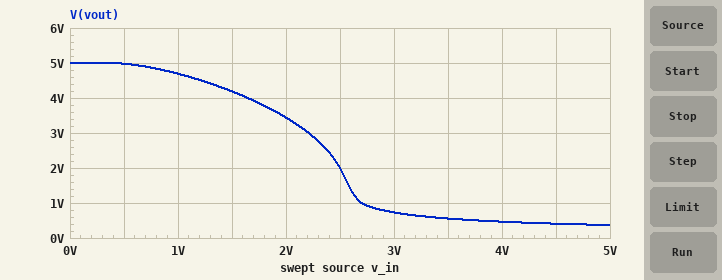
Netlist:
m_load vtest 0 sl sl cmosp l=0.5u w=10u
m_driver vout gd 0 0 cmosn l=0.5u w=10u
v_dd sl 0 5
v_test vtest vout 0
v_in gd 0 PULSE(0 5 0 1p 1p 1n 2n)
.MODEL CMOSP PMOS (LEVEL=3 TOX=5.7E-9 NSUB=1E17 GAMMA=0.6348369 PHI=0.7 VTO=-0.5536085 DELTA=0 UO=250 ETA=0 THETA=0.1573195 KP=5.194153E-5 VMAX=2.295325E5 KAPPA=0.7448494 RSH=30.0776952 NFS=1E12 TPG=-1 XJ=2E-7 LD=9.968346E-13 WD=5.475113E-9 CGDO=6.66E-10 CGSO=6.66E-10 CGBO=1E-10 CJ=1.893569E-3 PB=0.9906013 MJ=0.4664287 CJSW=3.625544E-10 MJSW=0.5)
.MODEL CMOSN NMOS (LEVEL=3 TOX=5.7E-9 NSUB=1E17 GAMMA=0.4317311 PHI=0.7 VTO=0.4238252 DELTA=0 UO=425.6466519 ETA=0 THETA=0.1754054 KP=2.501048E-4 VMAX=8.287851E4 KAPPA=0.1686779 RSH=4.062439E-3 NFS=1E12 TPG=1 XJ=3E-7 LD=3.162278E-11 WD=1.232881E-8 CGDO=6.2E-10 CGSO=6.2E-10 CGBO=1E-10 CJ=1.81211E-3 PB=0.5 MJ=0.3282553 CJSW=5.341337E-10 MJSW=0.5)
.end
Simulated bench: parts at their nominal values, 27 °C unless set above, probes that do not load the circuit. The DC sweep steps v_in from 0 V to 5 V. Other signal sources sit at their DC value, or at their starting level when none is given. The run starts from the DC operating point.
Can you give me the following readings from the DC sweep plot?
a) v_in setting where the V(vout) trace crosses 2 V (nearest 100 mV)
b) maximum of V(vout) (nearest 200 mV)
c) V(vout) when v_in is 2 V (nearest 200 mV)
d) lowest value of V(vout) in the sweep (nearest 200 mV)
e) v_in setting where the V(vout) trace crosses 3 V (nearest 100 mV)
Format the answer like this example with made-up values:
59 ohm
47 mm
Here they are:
2.5 V
5.0 V
3.4 V
400 mV
2.2 V
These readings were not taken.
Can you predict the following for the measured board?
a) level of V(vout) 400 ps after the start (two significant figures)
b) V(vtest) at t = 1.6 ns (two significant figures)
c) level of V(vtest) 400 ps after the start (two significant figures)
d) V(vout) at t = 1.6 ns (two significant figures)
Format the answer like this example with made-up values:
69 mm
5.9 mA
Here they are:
370 mV
5.0 V
370 mV
5.0 V
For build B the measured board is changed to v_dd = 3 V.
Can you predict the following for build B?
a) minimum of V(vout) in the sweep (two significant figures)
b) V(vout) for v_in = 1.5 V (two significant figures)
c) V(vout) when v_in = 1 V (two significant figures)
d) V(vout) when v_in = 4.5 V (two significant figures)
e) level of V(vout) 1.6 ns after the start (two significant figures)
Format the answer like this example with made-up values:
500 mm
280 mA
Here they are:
130 mV
1.4 V
2.6 V
140 mV
3.0 V
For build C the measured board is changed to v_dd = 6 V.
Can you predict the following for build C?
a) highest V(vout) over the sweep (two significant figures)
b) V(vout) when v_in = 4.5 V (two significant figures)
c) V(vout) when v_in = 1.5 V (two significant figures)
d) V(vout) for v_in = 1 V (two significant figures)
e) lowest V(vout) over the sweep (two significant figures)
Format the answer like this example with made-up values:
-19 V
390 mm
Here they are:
6.0 V
610 mV
5.3 V
5.7 V
540 mV
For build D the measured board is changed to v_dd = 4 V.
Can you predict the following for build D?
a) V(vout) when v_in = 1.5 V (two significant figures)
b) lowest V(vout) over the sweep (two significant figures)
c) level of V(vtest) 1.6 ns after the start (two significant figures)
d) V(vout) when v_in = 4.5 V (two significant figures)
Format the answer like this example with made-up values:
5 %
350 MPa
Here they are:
3.0 V
240 mV
4.0 V
260 mV
